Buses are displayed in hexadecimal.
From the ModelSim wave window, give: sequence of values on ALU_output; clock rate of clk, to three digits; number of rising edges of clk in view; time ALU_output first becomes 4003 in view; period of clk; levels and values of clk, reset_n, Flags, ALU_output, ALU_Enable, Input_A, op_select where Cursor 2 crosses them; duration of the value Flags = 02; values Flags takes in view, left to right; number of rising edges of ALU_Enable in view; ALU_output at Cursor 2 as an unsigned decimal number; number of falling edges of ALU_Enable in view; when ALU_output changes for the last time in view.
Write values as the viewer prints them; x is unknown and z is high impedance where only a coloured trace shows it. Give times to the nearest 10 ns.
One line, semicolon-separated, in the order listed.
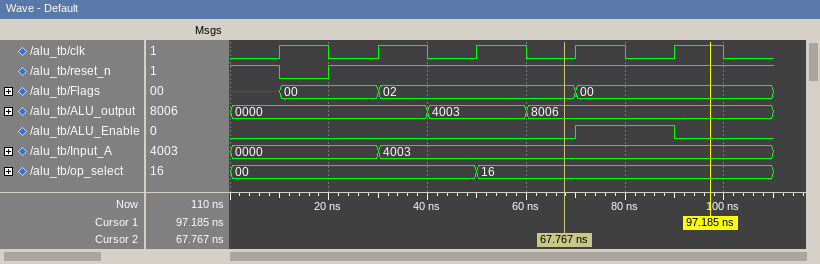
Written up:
0000, 4003, 8006; 50.0 MHz; 5; 40 ns; 20 ns; clk=0, reset_n=1, Flags=02, ALU_output=8006, ALU_Enable=0, Input_A=4003, op_select=16; 40 ns; x, 00, 02, 00; 1; 32774; 1; 60 ns
